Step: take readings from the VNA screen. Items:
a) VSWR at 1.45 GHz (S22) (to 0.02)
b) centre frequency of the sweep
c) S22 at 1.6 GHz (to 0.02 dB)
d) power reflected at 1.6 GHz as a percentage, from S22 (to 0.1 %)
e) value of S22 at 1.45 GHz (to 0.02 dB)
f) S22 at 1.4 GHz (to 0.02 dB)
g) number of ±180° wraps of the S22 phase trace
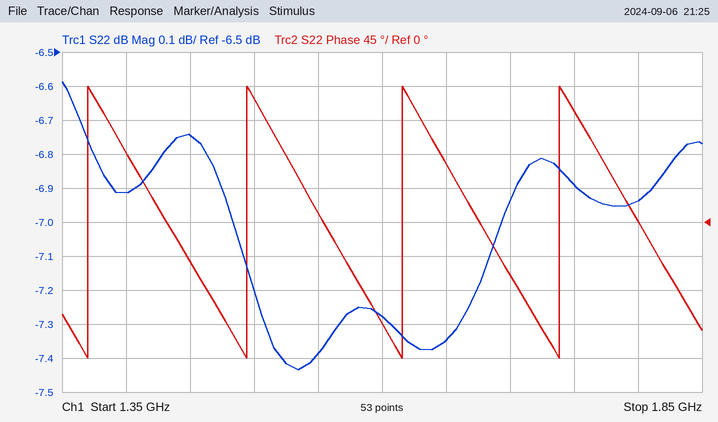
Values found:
2.70
1.6 GHz
-7.28 dB
18.7 %
-6.74 dB
-6.92 dB
4
